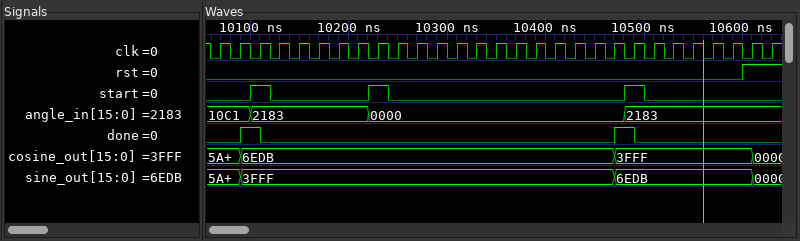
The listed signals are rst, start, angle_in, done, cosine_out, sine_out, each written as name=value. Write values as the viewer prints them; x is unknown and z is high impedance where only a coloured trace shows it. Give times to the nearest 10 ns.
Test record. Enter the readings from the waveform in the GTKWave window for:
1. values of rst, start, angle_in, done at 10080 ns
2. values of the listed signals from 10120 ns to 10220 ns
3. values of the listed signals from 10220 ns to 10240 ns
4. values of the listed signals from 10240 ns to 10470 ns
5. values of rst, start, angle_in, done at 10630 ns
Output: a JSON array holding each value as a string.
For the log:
["rst=0, start=0, angle_in=10C1, done=0", "rst=0, start=0, angle_in=2183, done=0, cosine_out=6EDB, sine_out=3FFF", "rst=0, start=1, angle_in=0000, done=0, cosine_out=6EDB, sine_out=3FFF", "rst=0, start=0, angle_in=0000, done=0, cosine_out=6EDB, sine_out=3FFF", "rst=1, start=0, angle_in=2183, done=0"]
